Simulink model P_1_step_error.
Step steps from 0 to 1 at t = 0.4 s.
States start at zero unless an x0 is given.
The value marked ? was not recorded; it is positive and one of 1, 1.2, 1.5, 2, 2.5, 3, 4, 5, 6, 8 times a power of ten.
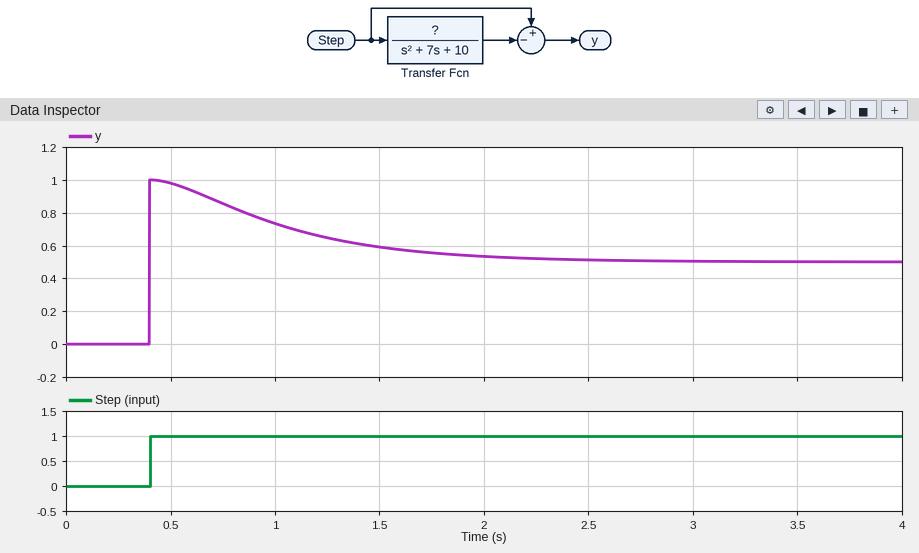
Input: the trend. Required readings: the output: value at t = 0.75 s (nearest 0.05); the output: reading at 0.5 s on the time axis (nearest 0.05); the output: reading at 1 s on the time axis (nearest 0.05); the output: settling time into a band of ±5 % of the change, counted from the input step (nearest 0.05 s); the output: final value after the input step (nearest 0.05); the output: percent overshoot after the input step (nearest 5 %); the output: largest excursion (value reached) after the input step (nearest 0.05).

0.85
1.00
0.75
1.75 s
0.50
100 %
1.00
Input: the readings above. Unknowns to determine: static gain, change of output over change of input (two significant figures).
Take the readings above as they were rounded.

0.50
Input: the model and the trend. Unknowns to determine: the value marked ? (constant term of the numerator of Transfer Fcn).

5
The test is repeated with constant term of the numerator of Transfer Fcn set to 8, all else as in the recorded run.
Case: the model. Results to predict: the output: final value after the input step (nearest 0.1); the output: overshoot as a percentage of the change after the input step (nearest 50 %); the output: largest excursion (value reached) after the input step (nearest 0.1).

0.2
400 %
1.0
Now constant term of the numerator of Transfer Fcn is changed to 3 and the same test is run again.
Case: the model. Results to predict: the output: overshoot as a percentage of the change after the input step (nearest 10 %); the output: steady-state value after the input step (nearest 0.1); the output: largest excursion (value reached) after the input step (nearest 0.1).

40 %
0.7
1.0
